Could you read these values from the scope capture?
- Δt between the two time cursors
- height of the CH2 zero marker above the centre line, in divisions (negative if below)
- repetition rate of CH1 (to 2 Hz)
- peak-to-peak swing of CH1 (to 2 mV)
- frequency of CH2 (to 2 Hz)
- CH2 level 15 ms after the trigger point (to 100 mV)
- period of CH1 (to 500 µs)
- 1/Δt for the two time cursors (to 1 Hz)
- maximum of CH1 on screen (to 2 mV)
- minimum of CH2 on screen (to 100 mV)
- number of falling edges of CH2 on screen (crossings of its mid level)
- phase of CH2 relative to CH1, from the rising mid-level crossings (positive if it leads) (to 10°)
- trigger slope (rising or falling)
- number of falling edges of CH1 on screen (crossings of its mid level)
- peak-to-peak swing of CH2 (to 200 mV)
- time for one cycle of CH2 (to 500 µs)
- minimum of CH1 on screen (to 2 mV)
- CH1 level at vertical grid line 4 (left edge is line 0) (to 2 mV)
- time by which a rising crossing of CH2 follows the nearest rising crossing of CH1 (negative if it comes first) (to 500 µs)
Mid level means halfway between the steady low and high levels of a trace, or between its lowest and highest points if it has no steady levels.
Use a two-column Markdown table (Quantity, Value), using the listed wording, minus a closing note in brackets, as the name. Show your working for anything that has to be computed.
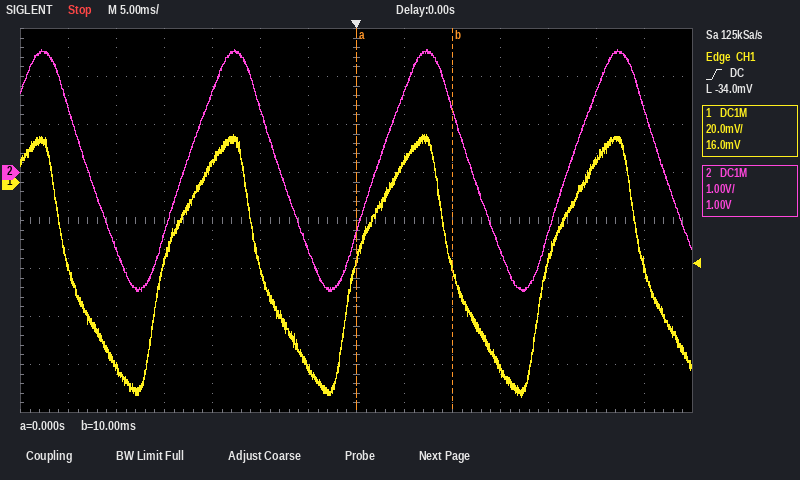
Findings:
| Quantity | Value |
|---|---|
| Δt between the two time cursors | 10 ms − (0 s) = 10.0 ms |
| height of the CH2 zero marker above the centre line, in divisions | +1.0 div |
| repetition rate of CH1 | 1 / 20.0 ms ≈ 50 Hz |
| peak-to-peak swing of CH1 | 20 mV − (-90 mV) = 110 mV |
| frequency of CH2 | 1 / 20.0 ms ≈ 50 Hz |
| CH2 level 15 ms after the trigger point | -1.6 V |
| period of CH1 | 20.0 ms |
| 1/Δt for the two time cursors | 1 / 10.0 ms ≈ 100 Hz |
| maximum of CH1 on screen | 20 mV |
| minimum of CH2 on screen | -2.5 V |
| number of falling edges of CH2 on screen | 4 |
| phase of CH2 relative to CH1, from the rising mid-level crossings (positive if it leads) | −360° × (+2.0 ms) / 20.0 ms ≈ -36.0°, so -40° to the nearest 10° |
| trigger slope | rising |
| number of falling edges of CH1 on screen | 4 |
| peak-to-peak swing of CH2 | 5.0 V |
| time for one cycle of CH2 | 20.0 ms |
| minimum of CH1 on screen | -90 mV |
| CH1 level at vertical grid line 4 (left edge is line 0) | 8 mV |
| time by which a rising crossing of CH2 follows the nearest rising crossing of CH1 (negative if it comes first) | +2.0 ms |
